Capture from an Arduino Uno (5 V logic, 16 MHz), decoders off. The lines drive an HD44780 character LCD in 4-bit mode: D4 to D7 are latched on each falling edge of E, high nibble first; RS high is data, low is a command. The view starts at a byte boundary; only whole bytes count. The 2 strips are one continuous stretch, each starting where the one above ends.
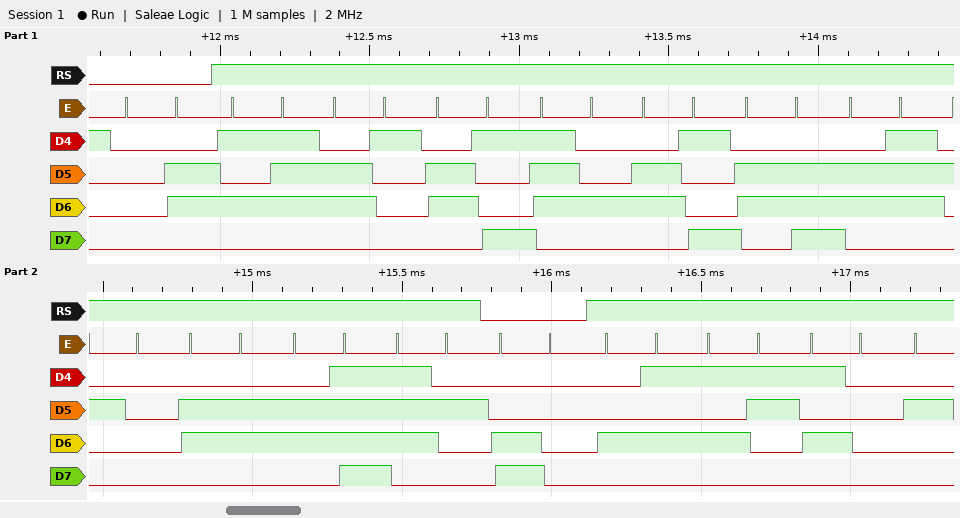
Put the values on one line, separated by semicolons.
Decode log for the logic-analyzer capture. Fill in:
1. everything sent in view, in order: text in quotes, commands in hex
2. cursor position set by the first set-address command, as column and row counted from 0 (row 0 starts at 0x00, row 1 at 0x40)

0x06 "Waiting for" 0xC0 "ESP"; column 0, row 1
